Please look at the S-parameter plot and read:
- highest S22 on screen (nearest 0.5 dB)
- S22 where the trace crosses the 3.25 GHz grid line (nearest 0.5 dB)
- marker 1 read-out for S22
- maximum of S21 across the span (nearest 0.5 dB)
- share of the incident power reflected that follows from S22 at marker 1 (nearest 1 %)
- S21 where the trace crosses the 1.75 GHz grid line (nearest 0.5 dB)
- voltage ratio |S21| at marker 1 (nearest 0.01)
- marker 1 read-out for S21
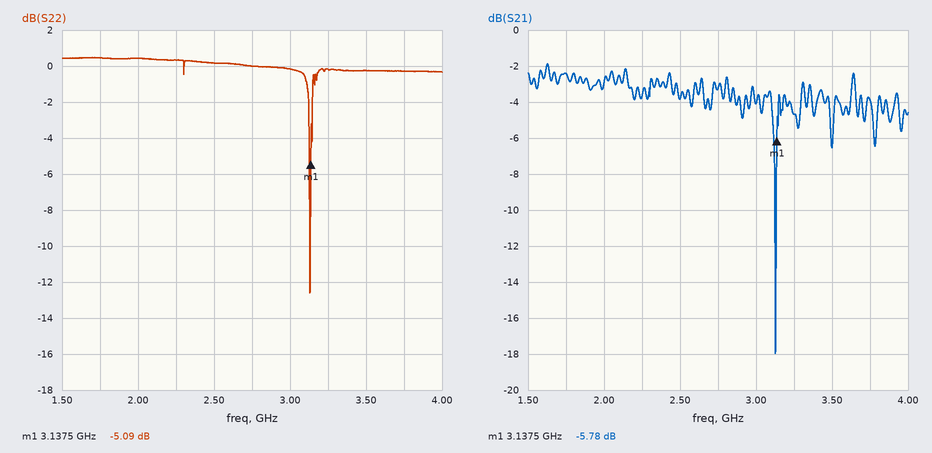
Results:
0.5 dB
0.0 dB
-5.09 dB
-2.0 dB
31 %
-2.5 dB
0.51
-5.78 dB
